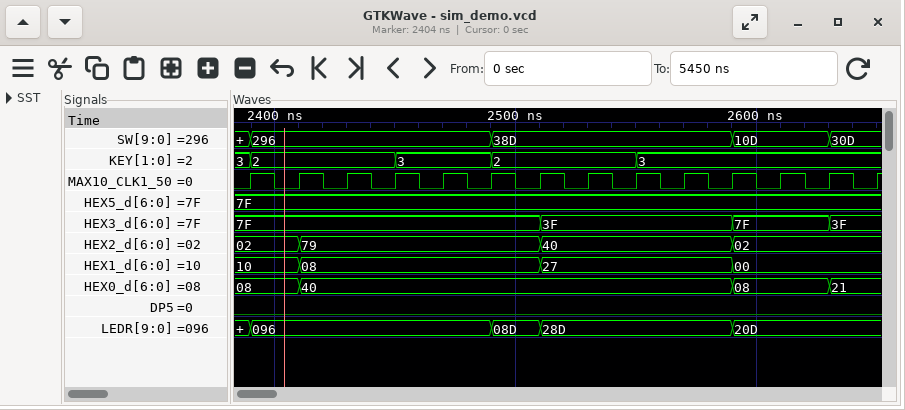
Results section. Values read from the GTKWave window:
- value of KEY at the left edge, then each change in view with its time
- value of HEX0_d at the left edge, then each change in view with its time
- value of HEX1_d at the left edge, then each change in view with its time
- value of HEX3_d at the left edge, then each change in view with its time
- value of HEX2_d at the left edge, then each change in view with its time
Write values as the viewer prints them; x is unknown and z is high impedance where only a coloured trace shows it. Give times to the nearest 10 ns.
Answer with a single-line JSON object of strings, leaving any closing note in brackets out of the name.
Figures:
{"value of KEY at the left edge, then each change in view with its time": "3, 2 at 2390 ns, 3 at 2450 ns, 2 at 2490 ns, 3 at 2550 ns", "value of HEX0_d at the left edge, then each change in view with its time": "08, 40 at 2410 ns, 08 at 2590 ns, 21 at 2630 ns", "value of HEX1_d at the left edge, then each change in view with its time": "10, 08 at 2410 ns, 27 at 2510 ns, 00 at 2590 ns", "value of HEX3_d at the left edge, then each change in view with its time": "7F, 3F at 2510 ns, 7F at 2590 ns, 3F at 2630 ns", "value of HEX2_d at the left edge, then each change in view with its time": "02, 79 at 2410 ns, 40 at 2510 ns, 02 at 2590 ns"}
